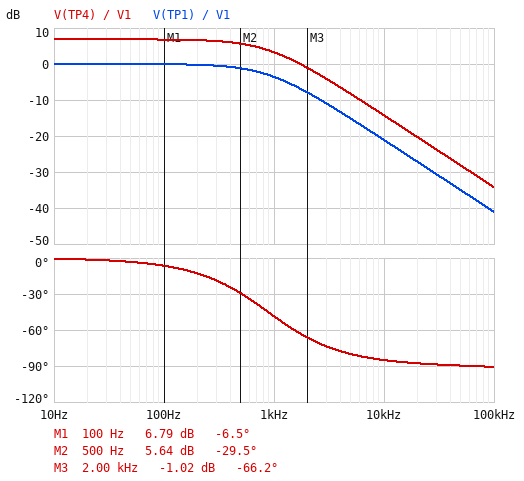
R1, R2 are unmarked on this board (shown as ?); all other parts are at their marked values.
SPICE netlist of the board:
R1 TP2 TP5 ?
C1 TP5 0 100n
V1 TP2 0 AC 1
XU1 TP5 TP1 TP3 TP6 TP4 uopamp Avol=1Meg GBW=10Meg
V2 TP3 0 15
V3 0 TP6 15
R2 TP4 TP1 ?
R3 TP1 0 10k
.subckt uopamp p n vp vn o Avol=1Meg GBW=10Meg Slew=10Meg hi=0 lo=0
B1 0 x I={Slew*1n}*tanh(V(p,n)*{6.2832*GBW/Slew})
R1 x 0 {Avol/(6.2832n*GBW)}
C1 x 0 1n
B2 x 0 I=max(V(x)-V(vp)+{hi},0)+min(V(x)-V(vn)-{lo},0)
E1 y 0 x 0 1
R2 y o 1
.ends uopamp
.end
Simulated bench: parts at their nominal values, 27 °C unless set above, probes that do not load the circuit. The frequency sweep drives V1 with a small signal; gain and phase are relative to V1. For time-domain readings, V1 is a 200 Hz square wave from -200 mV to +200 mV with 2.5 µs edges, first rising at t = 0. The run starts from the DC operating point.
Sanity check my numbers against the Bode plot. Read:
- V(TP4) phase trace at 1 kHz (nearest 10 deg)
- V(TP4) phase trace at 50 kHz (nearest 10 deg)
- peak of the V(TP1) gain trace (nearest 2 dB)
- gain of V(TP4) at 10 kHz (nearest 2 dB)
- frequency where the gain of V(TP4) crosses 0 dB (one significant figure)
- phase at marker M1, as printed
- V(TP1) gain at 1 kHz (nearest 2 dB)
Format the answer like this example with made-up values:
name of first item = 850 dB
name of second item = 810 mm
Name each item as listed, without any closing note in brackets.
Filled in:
V(TP4) phase trace at 1 kHz = -50 deg
V(TP4) phase trace at 50 kHz = -90 deg
peak of the V(TP1) gain trace = 0 dB
gain of V(TP4) at 10 kHz = -14 dB
frequency where the gain of V(TP4) crosses 0 dB = 2 kHz
phase at marker M1, as printed = -6.5 deg
V(TP1) gain at 1 kHz = -4 dB
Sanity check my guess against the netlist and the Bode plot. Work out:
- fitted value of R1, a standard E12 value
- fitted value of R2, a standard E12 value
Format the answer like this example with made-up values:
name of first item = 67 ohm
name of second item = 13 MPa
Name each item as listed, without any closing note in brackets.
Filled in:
fitted value of R1, a standard E12 value = 1.8 kΩ
fitted value of R2, a standard E12 value = 12 kΩ
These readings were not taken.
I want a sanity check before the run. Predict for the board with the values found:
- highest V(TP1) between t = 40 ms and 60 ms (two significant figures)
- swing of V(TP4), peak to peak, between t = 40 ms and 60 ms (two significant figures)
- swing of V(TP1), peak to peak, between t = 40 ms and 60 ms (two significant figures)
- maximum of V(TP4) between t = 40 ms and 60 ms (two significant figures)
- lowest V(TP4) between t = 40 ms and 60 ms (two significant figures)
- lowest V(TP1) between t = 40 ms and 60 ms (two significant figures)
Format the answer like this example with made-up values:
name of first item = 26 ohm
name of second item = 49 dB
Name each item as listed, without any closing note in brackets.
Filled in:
highest V(TP1) between t = 40 ms and 60 ms = 200 mV
swing of V(TP4), peak to peak, between t = 40 ms and 60 ms = 880 mV
swing of V(TP1), peak to peak, between t = 40 ms and 60 ms = 400 mV
maximum of V(TP4) between t = 40 ms and 60 ms = 440 mV
lowest V(TP4) between t = 40 ms and 60 ms = -440 mV
lowest V(TP1) between t = 40 ms and 60 ms = -200 mV
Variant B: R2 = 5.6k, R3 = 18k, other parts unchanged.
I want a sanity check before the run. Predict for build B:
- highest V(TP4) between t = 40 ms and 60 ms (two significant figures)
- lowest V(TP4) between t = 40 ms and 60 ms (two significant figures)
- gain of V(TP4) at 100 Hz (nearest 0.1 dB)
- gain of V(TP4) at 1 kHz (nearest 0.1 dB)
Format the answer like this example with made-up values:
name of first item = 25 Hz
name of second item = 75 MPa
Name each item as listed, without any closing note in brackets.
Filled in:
highest V(TP4) between t = 40 ms and 60 ms = 260 mV
lowest V(TP4) between t = 40 ms and 60 ms = -260 mV
gain of V(TP4) at 100 Hz = 2.3 dB
gain of V(TP4) at 1 kHz = -1.2 dB
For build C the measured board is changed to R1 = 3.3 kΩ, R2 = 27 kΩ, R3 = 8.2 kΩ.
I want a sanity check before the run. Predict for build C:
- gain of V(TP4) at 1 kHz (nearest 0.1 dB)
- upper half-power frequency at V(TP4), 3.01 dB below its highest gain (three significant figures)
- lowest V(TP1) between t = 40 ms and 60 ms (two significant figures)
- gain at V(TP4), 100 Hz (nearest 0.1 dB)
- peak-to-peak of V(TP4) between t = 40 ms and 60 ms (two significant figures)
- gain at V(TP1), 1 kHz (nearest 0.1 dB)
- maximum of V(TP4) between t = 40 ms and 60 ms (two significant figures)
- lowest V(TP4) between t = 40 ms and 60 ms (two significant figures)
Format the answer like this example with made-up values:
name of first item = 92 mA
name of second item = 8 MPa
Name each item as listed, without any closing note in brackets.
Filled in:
gain of V(TP4) at 1 kHz = 5.4 dB
upper half-power frequency at V(TP4), 3.01 dB below its highest gain = 482 Hz
lowest V(TP1) between t = 40 ms and 60 ms = -200 mV
gain at V(TP4), 100 Hz = 12.5 dB
peak-to-peak of V(TP4) between t = 40 ms and 60 ms = 1.7 V
gain at V(TP1), 1 kHz = -7.2 dB
maximum of V(TP4) between t = 40 ms and 60 ms = 860 mV
lowest V(TP4) between t = 40 ms and 60 ms = -860 mV
